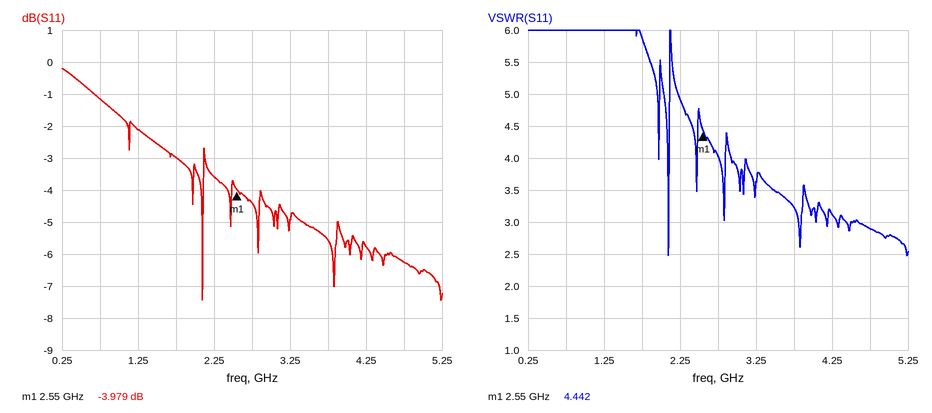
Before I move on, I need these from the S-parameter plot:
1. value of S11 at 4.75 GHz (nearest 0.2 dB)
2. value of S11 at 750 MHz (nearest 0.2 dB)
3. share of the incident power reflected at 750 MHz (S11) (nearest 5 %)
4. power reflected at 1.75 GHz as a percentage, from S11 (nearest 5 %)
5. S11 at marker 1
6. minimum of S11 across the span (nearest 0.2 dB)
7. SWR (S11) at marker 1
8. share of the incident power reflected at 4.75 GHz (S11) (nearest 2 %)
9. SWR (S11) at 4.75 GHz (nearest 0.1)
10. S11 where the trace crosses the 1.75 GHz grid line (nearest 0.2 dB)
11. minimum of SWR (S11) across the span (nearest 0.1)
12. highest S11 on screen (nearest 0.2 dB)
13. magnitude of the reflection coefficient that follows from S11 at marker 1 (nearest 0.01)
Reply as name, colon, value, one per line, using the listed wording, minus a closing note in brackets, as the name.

value of S11 at 4.75 GHz: -6.2 dB
value of S11 at 750 MHz: -1.2 dB
share of the incident power reflected at 750 MHz (S11): 75 %
power reflected at 1.75 GHz as a percentage, from S11: 50 %
S11 at marker 1: -3.979 dB
minimum of S11 across the span: -7.4 dB
SWR (S11) at marker 1: 4.442
share of the incident power reflected at 4.75 GHz (S11): 24 %
SWR (S11) at 4.75 GHz: 2.9
S11 where the trace crosses the 1.75 GHz grid line: -3.0 dB
minimum of SWR (S11) across the span: 2.5
highest S11 on screen: -0.2 dB
magnitude of the reflection coefficient that follows from S11 at marker 1: 0.63
